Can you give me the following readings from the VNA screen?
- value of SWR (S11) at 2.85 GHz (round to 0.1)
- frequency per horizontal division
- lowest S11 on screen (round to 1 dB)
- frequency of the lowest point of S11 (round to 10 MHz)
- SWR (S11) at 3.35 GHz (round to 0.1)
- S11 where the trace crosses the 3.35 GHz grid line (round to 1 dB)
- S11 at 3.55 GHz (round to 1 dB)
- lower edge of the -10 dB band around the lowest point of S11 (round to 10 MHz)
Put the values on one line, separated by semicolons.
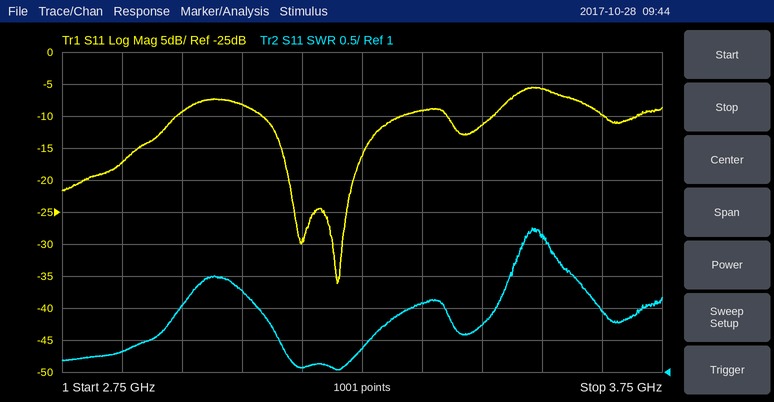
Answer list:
1.3; 100 MHz; -36 dB; 3.21 GHz; 2.1; -9 dB; -6 dB; 3.08 GHz
